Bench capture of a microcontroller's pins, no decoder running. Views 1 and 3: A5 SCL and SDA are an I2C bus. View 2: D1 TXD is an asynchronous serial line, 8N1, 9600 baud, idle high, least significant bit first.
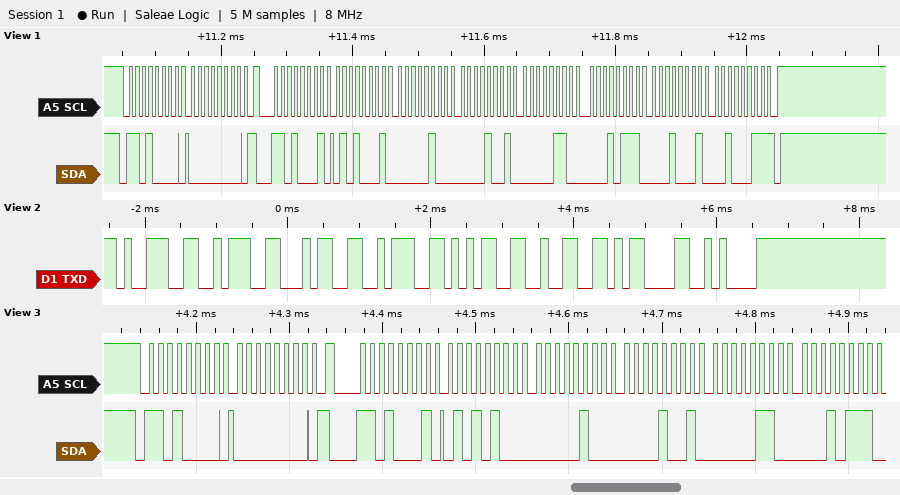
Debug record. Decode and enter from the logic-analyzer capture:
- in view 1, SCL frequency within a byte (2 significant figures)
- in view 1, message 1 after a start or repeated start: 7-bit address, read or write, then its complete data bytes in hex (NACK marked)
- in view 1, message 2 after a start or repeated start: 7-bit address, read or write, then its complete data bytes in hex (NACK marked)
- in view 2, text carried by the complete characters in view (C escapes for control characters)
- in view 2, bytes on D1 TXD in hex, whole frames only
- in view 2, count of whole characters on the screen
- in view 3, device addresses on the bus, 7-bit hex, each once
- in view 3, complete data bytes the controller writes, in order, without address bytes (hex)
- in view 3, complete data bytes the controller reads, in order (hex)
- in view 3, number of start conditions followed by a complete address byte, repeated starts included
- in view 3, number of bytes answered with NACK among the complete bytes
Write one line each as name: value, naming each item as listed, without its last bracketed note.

in view 1, SCL frequency within a byte: 100 kHz
in view 1, message 1 after a start or repeated start: 7-bit address, read or write, then its complete data bytes in hex: 0x68 write: 00
in view 1, message 2 after a start or repeated start: 7-bit address, read or write, then its complete data bytes in hex: 0x68 read: 51 04 09 06 17 11 23 NACK
in view 2, text carried by the complete characters in view: "9:4:52\r\n"
in view 2, bytes on D1 TXD in hex, whole frames only: 39 3A 34 3A 35 32 0D 0A
in view 2, count of whole characters on the screen: 8
in view 3, device addresses on the bus, 7-bit hex, each once: 0x68
in view 3, complete data bytes the controller writes, in order, without address bytes: 00
in view 3, complete data bytes the controller reads, in order: 54 04 09 06 17
in view 3, number of start conditions followed by a complete address byte, repeated starts included: 2
in view 3, number of bytes answered with NACK among the complete bytes: 0
